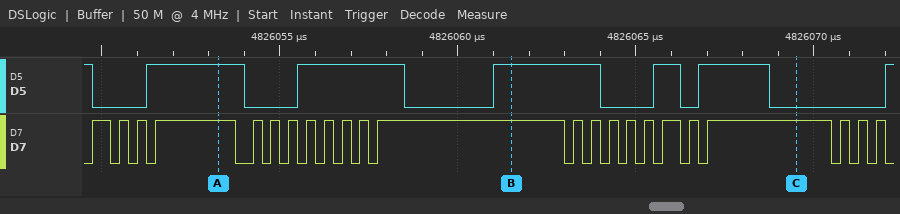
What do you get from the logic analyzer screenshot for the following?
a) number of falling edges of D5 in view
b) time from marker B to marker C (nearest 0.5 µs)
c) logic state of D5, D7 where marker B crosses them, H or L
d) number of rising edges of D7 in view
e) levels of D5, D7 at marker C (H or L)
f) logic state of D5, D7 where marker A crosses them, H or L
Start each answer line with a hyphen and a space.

- 6
- 8 µs
- D5=H, D7=H
- 23
- D5=L, D7=H
- D5=H, D7=H
